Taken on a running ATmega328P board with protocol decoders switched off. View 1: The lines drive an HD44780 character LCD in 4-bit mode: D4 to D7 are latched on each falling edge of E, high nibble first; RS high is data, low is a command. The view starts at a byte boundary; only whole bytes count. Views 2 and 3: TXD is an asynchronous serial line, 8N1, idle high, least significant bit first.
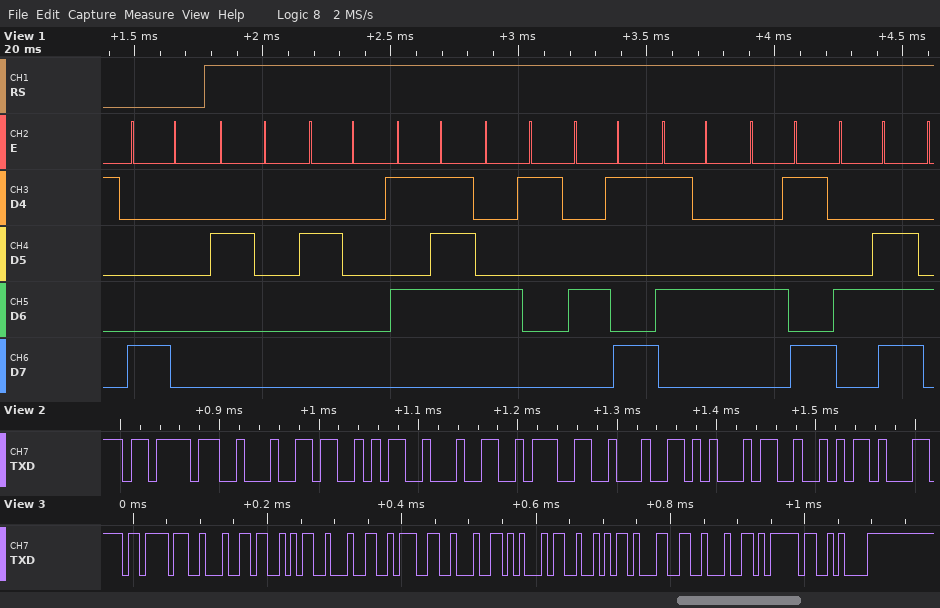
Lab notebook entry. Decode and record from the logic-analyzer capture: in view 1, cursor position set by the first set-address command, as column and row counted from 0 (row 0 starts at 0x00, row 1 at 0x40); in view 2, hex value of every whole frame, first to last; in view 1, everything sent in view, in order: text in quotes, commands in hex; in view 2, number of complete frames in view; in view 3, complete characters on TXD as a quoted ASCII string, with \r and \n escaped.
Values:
column 0, row 0
7B 22 53 22 3A 22 45 52
0x80 "  WAITIN"
8
"{\"S\":\"ER1\"}\n"
